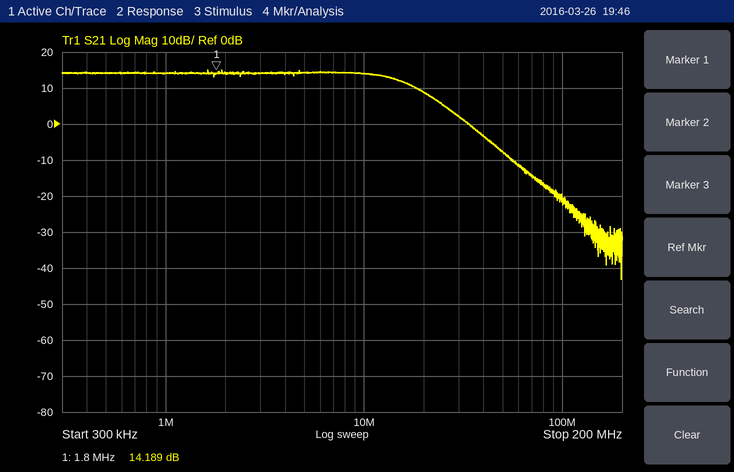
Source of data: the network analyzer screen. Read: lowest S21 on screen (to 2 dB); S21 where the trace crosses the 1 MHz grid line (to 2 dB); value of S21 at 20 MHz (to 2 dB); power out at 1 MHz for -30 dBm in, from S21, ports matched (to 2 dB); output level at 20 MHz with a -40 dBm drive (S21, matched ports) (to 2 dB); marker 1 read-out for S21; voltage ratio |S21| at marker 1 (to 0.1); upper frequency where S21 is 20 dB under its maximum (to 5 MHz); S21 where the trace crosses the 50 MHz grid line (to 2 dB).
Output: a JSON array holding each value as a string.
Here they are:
["-44 dB", "14 dB", "8 dB", "-16 dBm", "-32 dBm", "14.189 dB", "5.1", "45 MHz", "-8 dB"]
